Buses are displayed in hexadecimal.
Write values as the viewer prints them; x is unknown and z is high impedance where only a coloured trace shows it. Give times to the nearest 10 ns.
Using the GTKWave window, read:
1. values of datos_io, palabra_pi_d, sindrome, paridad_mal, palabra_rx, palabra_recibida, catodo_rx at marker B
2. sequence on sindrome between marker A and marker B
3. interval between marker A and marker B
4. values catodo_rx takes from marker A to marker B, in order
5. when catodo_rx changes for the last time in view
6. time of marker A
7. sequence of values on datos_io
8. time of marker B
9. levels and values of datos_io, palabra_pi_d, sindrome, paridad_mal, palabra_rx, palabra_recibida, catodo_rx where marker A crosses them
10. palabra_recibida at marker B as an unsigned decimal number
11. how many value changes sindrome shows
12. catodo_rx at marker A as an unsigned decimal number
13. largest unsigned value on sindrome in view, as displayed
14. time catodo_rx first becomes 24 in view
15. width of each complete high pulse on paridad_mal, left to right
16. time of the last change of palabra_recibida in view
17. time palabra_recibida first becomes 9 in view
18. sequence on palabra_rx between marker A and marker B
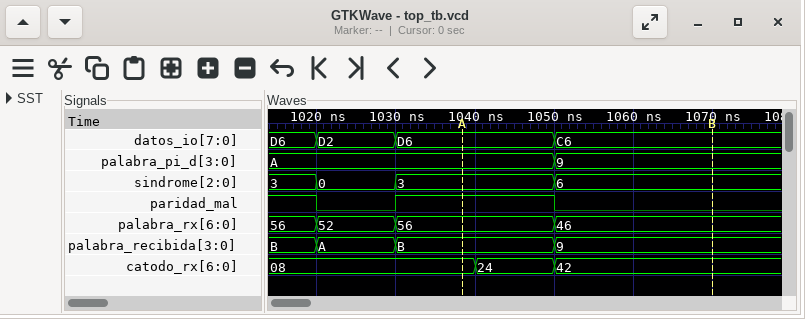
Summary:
datos_io=C6, palabra_pi_d=9, sindrome=6, paridad_mal=0, palabra_rx=46, palabra_recibida=9, catodo_rx=42
3, 6
30 ns
08, 24, 42
1050 ns
1040 ns
D6, D2, D6, C6
1070 ns
datos_io=D6, palabra_pi_d=A, sindrome=3, paridad_mal=1, palabra_rx=56, palabra_recibida=B, catodo_rx=08
9
3
8
6
1040 ns
20 ns
1050 ns
1050 ns
56, 46
